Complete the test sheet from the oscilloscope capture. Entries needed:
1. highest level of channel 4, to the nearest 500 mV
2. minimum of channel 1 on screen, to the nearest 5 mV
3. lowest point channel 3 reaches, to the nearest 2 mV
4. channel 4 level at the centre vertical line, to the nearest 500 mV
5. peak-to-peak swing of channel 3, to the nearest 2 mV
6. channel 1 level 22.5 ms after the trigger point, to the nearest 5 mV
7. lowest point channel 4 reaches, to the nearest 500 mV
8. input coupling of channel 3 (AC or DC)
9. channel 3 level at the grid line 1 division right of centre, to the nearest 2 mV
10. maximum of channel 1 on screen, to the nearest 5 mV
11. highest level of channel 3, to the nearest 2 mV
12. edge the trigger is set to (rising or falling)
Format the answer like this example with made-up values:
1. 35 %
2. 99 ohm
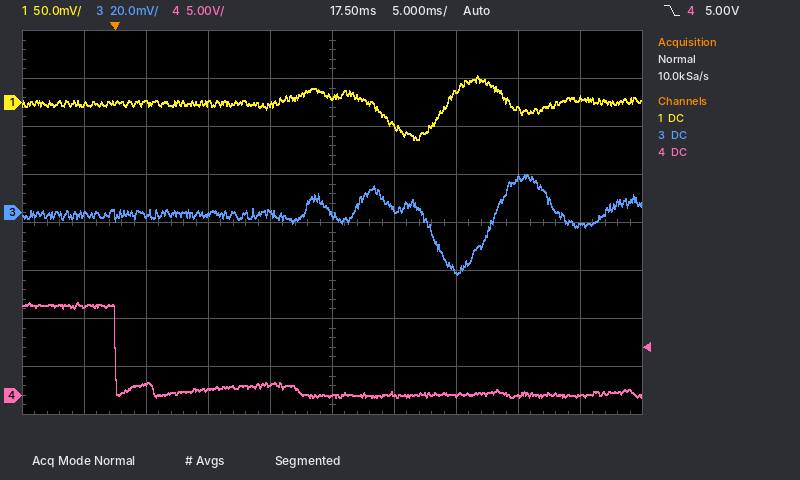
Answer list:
1. 9.5 V
2. -40 mV
3. -26 mV
4. 0.0 V
5. 42 mV
6. -25 mV
7. 0.0 V
8. DC
9. 2 mV
10. 30 mV
11. 16 mV
12. falling
